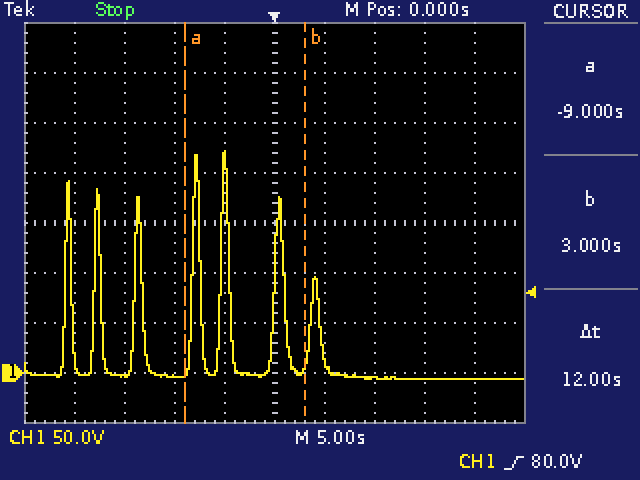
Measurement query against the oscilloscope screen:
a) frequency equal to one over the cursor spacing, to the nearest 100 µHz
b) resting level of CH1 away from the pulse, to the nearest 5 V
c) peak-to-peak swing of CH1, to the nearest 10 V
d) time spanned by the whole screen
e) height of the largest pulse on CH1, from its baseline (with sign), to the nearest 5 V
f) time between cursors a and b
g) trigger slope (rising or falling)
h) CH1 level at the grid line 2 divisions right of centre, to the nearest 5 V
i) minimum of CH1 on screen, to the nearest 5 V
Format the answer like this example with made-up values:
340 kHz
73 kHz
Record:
83.3 mHz
-5 V
230 V
50 s
+225 V
12 s
rising
-5 V
-5 V
